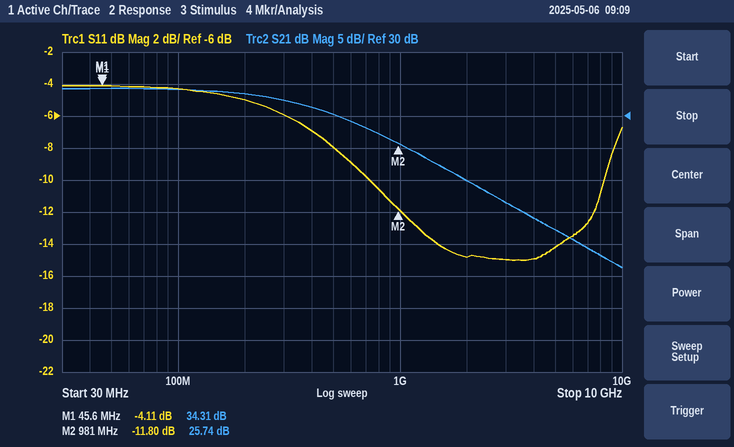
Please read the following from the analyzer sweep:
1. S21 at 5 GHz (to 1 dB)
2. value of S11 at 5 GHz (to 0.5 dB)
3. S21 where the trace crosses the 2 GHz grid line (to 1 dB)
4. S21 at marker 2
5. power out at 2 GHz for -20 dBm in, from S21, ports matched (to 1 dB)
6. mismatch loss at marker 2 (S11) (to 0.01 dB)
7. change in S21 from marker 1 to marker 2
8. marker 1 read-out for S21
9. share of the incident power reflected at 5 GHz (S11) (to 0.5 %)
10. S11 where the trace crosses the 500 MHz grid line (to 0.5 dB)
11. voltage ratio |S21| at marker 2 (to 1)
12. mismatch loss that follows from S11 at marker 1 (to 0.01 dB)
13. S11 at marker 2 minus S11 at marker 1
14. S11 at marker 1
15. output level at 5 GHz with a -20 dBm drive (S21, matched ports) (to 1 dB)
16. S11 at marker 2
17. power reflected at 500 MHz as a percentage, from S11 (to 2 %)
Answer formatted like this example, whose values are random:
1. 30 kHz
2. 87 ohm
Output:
1. 12 dB
2. -14.0 dB
3. 20 dB
4. 25.74 dB
5. 0 dBm
6. 0.30 dB
7. -8.57 dB
8. 34.31 dB
9. 4.0 %
10. -8.0 dB
11. 19
12. 2.13 dB
13. -7.69 dB
14. -4.11 dB
15. -8 dBm
16. -11.80 dB
17. 16 %
